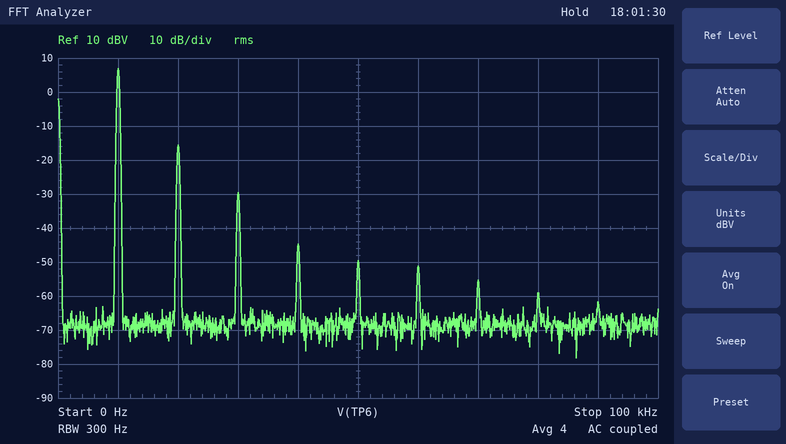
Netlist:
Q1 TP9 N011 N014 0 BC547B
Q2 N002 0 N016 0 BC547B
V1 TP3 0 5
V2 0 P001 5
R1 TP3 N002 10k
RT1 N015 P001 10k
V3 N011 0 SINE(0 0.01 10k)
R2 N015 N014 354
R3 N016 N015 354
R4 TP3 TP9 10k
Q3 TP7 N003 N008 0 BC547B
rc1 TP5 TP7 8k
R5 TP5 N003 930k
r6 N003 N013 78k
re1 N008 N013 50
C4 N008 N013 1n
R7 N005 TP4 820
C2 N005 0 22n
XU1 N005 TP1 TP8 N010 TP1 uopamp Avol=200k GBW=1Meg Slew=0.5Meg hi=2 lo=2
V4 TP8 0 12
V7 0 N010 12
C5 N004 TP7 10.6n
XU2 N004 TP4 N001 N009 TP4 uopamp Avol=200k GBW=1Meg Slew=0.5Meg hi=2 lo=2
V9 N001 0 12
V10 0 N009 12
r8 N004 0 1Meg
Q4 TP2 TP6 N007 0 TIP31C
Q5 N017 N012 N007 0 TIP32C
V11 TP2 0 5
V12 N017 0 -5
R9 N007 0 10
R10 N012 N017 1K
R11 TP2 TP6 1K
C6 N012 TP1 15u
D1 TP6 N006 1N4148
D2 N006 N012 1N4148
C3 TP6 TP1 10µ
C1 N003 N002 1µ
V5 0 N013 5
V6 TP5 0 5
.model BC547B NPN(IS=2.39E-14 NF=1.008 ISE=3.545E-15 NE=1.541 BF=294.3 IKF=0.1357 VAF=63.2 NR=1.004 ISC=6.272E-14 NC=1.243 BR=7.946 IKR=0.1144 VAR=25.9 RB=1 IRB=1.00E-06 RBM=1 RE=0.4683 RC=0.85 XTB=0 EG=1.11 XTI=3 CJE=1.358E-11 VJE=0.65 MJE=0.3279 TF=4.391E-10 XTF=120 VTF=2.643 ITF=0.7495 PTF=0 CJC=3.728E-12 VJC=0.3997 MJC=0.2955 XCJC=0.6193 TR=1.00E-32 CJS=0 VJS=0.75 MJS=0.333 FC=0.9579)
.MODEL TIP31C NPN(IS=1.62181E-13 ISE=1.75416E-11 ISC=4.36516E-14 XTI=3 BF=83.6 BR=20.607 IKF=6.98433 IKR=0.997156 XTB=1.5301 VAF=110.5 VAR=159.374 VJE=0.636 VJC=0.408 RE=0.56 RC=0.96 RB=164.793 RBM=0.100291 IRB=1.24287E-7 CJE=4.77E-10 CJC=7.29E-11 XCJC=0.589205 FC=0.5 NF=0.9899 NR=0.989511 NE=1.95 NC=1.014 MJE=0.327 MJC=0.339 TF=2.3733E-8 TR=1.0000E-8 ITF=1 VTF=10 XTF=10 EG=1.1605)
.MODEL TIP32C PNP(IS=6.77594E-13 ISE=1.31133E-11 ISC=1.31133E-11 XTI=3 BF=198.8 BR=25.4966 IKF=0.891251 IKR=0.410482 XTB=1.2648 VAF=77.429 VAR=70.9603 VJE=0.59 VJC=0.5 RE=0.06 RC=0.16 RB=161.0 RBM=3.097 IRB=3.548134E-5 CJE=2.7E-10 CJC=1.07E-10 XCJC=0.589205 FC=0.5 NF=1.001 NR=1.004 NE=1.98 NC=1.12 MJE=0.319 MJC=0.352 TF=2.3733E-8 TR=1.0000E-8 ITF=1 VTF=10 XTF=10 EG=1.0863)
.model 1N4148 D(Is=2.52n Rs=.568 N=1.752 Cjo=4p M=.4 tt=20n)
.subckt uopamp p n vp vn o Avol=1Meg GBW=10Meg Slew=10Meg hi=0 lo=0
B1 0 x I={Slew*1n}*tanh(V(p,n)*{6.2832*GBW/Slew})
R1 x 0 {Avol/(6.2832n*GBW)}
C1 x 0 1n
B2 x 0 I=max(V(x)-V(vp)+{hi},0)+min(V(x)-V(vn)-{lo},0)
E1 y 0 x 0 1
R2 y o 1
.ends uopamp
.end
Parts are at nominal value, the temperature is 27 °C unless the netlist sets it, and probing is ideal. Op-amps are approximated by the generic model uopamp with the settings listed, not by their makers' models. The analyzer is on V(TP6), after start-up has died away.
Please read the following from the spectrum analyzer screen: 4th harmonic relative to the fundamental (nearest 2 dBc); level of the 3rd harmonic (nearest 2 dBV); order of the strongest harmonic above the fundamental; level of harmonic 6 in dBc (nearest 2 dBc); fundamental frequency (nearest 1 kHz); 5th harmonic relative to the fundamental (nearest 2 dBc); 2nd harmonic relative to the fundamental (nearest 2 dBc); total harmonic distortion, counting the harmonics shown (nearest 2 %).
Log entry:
-52 dBc
-30 dBV
2
-58 dBc
10 kHz
-56 dBc
-22 dBc
8 %
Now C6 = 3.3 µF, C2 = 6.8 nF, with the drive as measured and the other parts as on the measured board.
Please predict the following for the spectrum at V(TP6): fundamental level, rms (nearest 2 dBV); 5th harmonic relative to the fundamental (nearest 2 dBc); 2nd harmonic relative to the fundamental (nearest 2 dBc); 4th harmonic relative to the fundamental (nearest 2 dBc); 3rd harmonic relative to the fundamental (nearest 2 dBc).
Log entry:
10 dBV
-50 dBc
-20 dBc
-46 dBc
-32 dBc
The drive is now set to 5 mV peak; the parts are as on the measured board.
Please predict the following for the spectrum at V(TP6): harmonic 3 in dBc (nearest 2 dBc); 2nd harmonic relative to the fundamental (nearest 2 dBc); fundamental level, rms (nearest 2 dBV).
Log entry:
-50 dBc
-30 dBc
2 dBV
